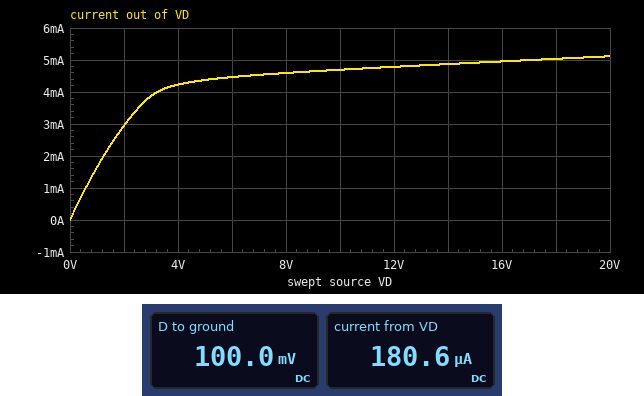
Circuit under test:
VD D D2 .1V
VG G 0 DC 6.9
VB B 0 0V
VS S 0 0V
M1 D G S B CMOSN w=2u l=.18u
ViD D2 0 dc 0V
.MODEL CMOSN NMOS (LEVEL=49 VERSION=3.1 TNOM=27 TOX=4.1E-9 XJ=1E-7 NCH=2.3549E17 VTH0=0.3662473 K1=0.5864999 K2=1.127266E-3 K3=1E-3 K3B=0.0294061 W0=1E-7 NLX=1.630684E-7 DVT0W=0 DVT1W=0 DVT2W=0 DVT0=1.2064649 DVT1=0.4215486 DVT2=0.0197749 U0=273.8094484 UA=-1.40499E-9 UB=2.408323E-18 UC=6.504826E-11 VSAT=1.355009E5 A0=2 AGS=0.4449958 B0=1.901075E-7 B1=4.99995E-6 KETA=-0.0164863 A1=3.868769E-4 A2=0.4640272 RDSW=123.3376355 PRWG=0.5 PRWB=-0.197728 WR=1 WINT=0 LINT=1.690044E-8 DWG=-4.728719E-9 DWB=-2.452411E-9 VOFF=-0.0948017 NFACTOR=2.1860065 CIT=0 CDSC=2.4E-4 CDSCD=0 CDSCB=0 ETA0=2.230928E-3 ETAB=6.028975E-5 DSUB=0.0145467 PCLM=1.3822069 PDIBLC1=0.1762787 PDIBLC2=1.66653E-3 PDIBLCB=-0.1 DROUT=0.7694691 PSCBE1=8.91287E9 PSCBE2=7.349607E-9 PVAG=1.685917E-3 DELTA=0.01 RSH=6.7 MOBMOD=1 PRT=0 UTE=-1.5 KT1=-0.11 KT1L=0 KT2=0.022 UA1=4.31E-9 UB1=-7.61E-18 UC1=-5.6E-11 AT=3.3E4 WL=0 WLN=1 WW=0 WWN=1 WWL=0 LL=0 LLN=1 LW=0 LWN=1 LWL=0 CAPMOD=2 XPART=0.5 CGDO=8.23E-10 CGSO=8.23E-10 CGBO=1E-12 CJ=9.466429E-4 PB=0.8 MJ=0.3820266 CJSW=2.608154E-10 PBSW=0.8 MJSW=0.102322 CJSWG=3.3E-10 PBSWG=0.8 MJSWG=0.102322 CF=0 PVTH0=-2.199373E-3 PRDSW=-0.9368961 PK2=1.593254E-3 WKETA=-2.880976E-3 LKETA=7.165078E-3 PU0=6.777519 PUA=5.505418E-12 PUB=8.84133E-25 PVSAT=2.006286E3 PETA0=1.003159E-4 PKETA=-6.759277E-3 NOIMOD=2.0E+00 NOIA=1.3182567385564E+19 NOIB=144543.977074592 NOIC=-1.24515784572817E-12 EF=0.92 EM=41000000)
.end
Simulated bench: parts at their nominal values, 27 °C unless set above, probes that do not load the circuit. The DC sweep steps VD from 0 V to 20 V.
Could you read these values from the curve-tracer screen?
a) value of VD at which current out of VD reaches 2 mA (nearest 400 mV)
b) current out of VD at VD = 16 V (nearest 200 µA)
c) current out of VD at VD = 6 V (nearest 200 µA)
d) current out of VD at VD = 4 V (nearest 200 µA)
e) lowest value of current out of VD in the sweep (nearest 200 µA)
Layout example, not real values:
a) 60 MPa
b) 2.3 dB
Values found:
a) 1.2 V
b) 5.0 mA
c) 4.4 mA
d) 4.2 mA
e) 0 A
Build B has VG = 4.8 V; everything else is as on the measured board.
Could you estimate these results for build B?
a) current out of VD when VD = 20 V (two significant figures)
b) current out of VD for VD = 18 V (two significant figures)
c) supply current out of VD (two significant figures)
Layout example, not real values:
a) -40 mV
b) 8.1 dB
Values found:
a) 4.0 mA
b) 3.9 mA
c) 230 µA
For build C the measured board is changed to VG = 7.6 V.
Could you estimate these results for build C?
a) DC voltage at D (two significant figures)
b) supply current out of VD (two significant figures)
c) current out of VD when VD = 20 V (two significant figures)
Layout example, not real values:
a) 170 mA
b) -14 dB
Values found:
a) 100 mV
b) 170 µA
c) 5.4 mA
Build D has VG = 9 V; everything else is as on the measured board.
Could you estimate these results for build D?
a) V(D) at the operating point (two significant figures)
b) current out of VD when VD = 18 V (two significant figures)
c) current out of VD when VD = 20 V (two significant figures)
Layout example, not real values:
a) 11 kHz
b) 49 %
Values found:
a) 100 mV
b) 5.9 mA
c) 6.0 mA
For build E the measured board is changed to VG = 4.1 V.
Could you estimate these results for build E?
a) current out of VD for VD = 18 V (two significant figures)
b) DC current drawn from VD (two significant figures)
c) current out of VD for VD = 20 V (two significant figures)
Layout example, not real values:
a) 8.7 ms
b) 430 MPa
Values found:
a) 3.5 mA
b) 260 µA
c) 3.6 mA
